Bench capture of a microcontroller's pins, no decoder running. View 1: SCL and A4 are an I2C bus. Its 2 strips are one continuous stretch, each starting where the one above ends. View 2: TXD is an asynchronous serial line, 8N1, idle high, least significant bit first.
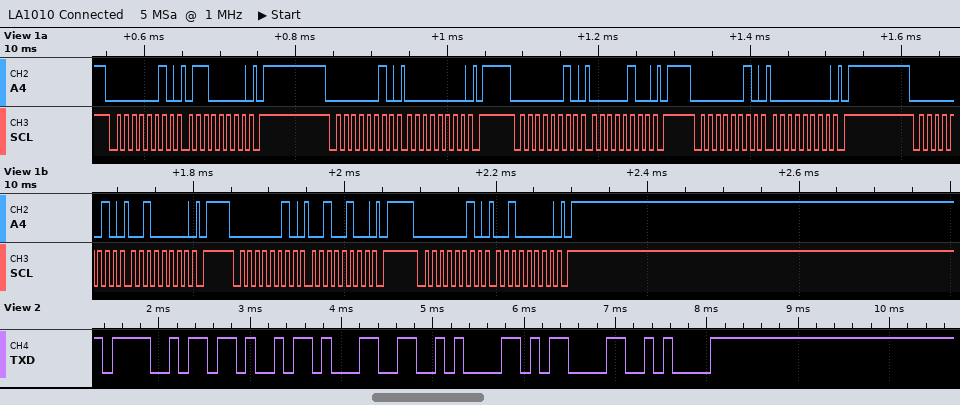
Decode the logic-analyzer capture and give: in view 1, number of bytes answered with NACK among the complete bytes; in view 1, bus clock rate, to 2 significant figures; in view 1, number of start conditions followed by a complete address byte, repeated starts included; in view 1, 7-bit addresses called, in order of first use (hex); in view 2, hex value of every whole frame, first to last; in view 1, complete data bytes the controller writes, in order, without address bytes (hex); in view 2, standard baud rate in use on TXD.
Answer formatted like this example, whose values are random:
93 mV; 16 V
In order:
0; 100 kHz; 7; 0x01; 0x4F 0x4B 0x31 0x0A 0x0D 0x0A; 60 00 04 00 20 24 20; 9600 baud
